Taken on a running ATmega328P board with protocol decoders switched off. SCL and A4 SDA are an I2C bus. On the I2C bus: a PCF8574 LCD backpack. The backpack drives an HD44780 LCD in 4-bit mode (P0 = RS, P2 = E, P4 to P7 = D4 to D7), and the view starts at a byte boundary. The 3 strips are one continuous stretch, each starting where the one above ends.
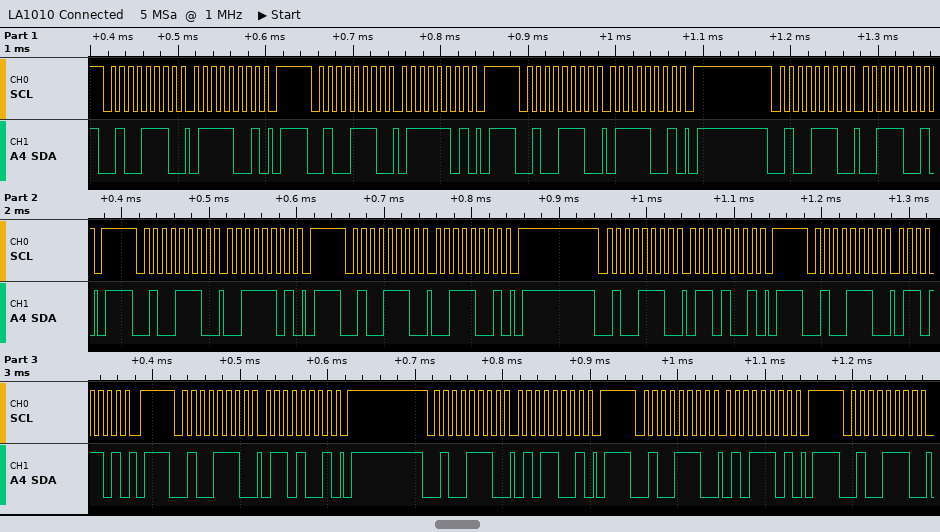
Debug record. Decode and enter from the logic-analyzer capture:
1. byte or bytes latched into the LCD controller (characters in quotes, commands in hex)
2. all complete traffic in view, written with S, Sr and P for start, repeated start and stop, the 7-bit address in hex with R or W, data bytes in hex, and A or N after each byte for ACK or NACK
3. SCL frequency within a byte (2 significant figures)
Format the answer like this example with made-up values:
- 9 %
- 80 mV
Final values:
- 's'
- S 27W A 79 A P S 27W A 7D A P S 27W A 79 A P S 27W A 39 A P S 27W A 3D A P S 27W A 39 A P S 27W A 69 A P S 27W A 6D A P S 27W A 69 A P S 27W A 59 A P S 27W A 5D A P S 27W A
- 100 kHz
